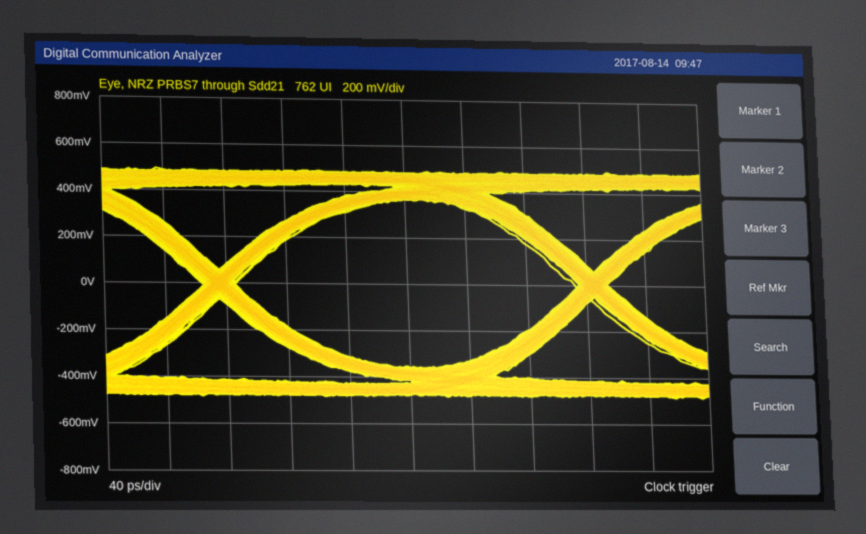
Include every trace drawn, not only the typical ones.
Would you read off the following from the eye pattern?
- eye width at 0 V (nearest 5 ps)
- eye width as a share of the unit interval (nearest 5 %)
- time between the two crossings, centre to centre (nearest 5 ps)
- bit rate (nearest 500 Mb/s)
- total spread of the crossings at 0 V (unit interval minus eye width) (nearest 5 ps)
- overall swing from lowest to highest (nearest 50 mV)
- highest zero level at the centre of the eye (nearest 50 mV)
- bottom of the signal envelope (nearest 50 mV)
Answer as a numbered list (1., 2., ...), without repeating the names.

1. 225 ps
2. 90 %
3. 250 ps
4. 4.0 Gb/s
5. 25 ps
6. 1.00 V
7. -350 mV
8. -500 mV
